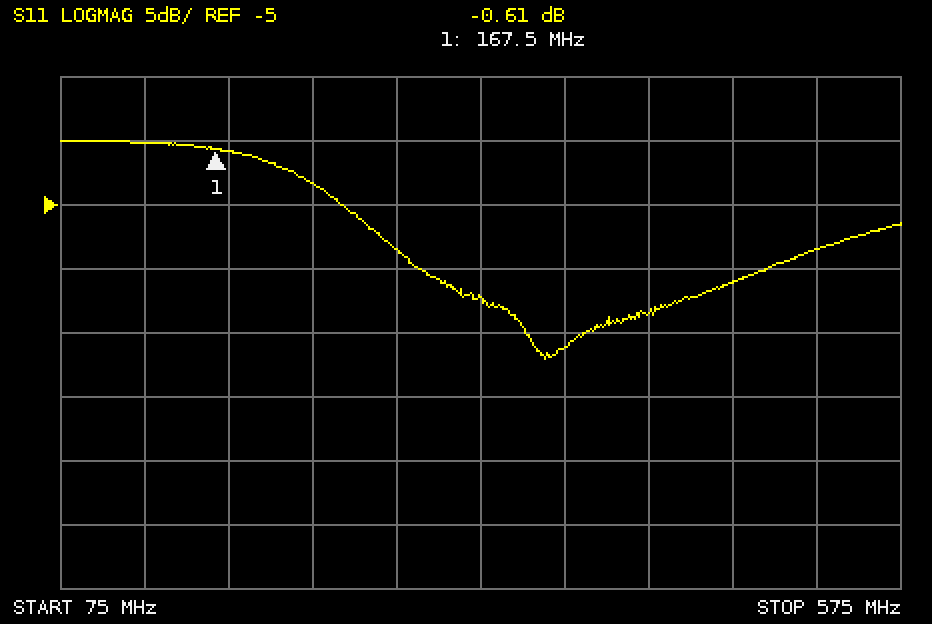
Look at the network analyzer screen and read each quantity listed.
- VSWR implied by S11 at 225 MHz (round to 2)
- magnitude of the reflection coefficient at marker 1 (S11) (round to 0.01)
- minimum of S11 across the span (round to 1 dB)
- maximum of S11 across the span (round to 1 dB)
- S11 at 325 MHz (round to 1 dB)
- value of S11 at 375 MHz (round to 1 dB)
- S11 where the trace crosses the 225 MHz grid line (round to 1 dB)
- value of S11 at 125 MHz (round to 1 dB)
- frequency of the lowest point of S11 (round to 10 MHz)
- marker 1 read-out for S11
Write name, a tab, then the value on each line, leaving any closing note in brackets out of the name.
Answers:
VSWR implied by S11 at 225 MHz	6
magnitude of the reflection coefficient at marker 1 (S11)	0.93
minimum of S11 across the span	-17 dB
maximum of S11 across the span	0 dB
S11 at 325 MHz	-12 dB
value of S11 at 375 MHz	-16 dB
S11 where the trace crosses the 225 MHz grid line	-3 dB
value of S11 at 125 MHz	0 dB
frequency of the lowest point of S11	360 MHz
marker 1 read-out for S11	-0.61 dB
